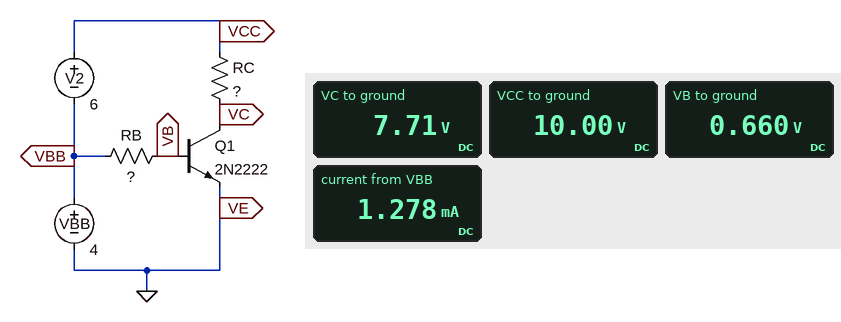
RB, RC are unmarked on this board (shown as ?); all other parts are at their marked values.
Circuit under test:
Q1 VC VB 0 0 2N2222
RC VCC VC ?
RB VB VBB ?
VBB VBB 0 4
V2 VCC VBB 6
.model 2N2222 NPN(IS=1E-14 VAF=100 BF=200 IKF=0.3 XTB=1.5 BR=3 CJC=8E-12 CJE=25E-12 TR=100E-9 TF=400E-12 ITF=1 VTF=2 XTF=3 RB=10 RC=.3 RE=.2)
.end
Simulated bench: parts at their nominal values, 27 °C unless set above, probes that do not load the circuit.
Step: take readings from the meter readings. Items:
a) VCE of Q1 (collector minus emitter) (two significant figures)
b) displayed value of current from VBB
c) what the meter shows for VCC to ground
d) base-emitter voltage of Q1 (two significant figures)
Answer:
7.7 V
1.278 mA
10.00 V
660 mV
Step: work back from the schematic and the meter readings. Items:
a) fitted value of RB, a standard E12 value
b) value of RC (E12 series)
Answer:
560 kΩ
1.8 kΩ
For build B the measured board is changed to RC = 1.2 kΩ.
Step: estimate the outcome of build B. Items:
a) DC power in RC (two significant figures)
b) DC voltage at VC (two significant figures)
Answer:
2.0 mW
8.5 V
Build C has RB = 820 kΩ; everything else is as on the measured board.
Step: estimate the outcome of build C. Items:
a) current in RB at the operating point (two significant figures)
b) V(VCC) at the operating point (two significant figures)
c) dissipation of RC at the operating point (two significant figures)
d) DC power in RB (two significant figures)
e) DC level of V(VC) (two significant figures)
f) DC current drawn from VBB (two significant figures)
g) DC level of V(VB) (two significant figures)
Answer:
4.1 µA
10 V
1.4 mW
14 µW
8.4 V
880 µA
650 mV
